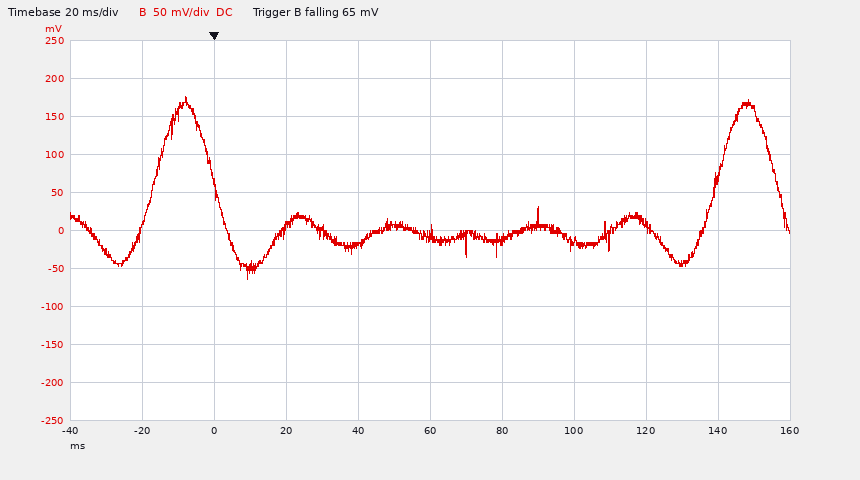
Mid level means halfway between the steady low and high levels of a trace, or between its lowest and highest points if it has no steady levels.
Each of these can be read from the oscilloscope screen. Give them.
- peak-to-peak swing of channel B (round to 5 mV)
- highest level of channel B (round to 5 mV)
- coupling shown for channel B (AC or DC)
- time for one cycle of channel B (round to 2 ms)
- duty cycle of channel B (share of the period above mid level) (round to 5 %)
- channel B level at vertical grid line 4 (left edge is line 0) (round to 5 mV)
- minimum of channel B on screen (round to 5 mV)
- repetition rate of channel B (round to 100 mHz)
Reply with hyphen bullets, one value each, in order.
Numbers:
- 240 mV
- 175 mV
- DC
- 156 ms
- 10 %
- -20 mV
- -65 mV
- 6.4 Hz
